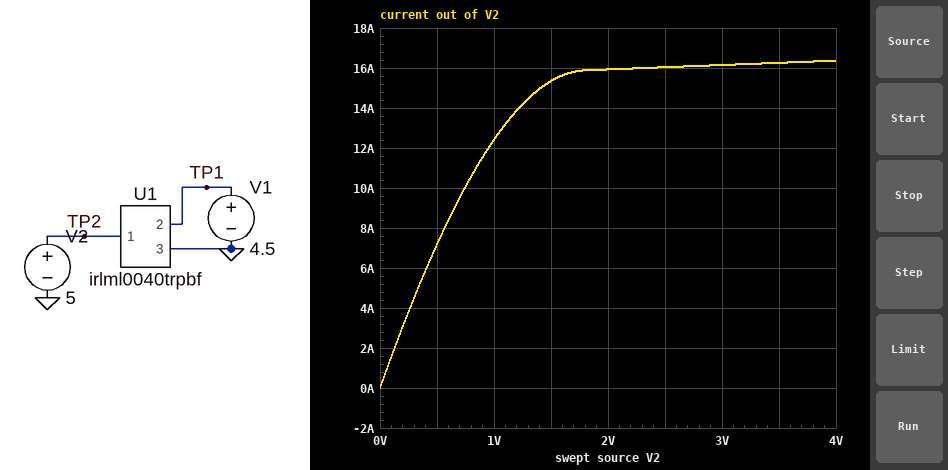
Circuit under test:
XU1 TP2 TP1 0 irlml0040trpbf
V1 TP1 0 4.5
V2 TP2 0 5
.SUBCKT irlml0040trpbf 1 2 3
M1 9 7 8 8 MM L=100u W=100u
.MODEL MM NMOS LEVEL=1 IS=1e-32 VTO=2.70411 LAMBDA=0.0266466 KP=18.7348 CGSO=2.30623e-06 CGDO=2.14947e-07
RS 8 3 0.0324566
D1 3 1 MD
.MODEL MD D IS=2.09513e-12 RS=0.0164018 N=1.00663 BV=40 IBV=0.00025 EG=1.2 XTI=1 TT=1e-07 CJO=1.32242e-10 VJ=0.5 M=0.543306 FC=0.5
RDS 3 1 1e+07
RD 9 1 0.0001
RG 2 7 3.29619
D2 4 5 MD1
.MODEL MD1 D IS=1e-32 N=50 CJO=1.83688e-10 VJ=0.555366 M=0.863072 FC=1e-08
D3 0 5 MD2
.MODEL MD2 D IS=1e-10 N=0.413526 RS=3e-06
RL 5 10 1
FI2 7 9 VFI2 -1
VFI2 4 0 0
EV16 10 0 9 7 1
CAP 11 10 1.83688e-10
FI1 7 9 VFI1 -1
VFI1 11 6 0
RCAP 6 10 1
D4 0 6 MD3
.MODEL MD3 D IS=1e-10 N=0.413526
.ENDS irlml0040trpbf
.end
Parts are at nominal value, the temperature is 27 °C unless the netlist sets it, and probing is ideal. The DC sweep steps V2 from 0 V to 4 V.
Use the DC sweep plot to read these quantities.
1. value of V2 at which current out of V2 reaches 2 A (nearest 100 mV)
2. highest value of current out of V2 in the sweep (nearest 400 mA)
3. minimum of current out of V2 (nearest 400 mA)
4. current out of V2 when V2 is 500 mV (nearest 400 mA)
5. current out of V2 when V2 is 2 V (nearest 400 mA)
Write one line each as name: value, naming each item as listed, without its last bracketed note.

value of V2 at which current out of V2 reaches 2 A: 100 mV
highest value of current out of V2 in the sweep: 16.4 A
minimum of current out of V2: 0 A
current out of V2 when V2 is 500 mV: 7.2 A
current out of V2 when V2 is 2 V: 16.0 A
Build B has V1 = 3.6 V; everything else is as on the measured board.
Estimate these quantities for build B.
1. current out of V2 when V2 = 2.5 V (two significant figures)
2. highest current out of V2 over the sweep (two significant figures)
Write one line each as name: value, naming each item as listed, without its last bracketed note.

current out of V2 when V2 = 2.5 V: 5.2 A
highest current out of V2 over the sweep: 5.4 A
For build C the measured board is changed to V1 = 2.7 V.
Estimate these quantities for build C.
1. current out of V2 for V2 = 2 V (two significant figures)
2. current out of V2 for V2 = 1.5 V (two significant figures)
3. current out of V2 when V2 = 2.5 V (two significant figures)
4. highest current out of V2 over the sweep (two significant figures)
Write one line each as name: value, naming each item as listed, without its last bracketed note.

current out of V2 for V2 = 2 V: 200 nA
current out of V2 for V2 = 1.5 V: 150 nA
current out of V2 when V2 = 2.5 V: 250 nA
highest current out of V2 over the sweep: 400 nA
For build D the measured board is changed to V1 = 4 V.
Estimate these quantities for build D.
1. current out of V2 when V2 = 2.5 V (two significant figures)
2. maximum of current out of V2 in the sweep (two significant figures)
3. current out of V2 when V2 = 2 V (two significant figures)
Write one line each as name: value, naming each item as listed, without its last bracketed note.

current out of V2 when V2 = 2.5 V: 9.6 A
maximum of current out of V2 in the sweep: 9.8 A
current out of V2 when V2 = 2 V: 9.5 A
